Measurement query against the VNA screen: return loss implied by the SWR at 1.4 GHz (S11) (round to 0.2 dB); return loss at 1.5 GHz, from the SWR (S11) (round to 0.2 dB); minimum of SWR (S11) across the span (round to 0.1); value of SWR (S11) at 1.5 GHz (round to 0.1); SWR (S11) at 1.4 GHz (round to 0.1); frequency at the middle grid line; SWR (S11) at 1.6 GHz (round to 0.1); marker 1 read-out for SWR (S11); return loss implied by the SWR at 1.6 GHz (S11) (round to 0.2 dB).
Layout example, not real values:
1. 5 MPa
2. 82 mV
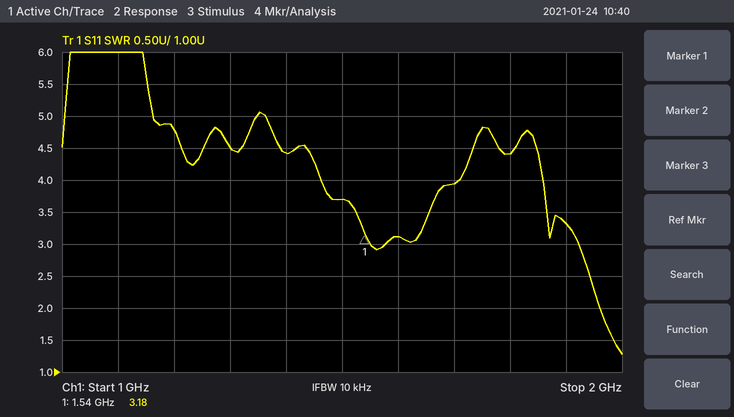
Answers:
1. 4.0 dB
2. 4.8 dB
3. 1.3
4. 3.7
5. 4.4
6. 1.5 GHz
7. 3.1
8. 3.18
9. 5.8 dB
